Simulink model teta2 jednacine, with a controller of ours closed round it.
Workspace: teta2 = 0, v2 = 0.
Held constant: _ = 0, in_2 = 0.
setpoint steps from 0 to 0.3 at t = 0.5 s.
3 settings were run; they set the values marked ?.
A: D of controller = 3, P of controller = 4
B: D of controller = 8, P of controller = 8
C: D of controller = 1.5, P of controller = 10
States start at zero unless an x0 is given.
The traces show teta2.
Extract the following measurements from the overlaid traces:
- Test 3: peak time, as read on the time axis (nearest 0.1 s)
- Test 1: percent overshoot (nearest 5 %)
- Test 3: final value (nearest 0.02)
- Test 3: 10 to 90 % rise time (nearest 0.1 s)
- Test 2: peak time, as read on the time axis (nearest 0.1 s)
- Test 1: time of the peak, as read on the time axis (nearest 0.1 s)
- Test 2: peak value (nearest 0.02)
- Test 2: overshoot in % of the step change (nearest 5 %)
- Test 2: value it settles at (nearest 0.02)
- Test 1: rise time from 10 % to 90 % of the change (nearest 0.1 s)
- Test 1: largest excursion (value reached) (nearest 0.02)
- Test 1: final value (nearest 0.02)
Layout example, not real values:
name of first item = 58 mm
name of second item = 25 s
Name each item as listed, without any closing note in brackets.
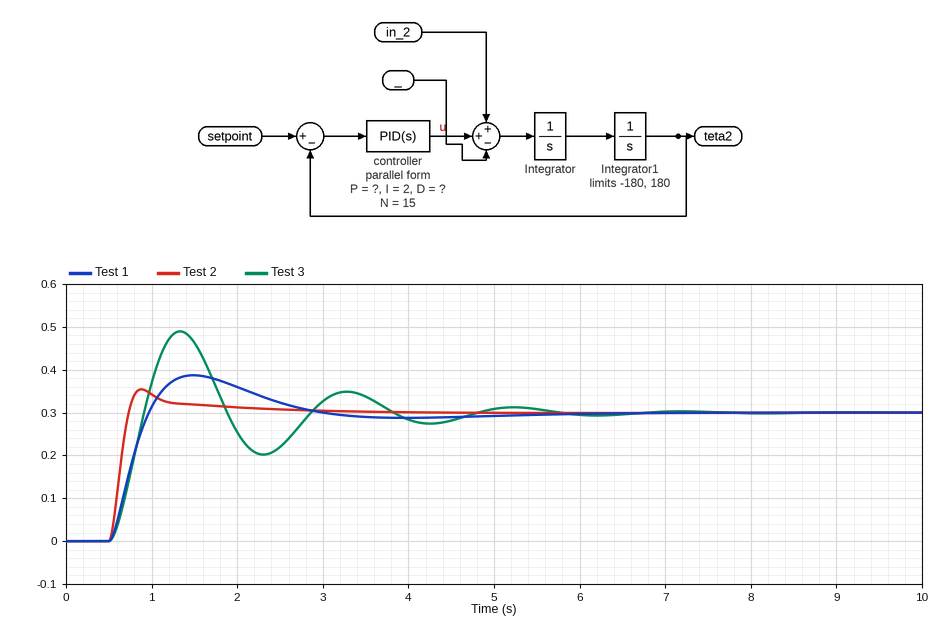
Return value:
Test 3: peak time, as read on the time axis = 1.3 s
Test 1: percent overshoot = 30 %
Test 3: final value = 0.30
Test 3: 10 to 90 % rise time = 0.3 s
Test 2: peak time, as read on the time axis = 0.9 s
Test 1: time of the peak, as read on the time axis = 1.5 s
Test 2: peak value = 0.36
Test 2: overshoot in % of the step change = 20 %
Test 2: value it settles at = 0.30
Test 1: rise time from 10 % to 90 % of the change = 0.3 s
Test 1: largest excursion (value reached) = 0.38
Test 1: final value = 0.30
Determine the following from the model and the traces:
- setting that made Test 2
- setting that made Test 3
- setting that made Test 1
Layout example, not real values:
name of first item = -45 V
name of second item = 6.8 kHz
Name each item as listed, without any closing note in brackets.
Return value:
setting that made Test 2 = B
setting that made Test 3 = C
setting that made Test 1 = A
